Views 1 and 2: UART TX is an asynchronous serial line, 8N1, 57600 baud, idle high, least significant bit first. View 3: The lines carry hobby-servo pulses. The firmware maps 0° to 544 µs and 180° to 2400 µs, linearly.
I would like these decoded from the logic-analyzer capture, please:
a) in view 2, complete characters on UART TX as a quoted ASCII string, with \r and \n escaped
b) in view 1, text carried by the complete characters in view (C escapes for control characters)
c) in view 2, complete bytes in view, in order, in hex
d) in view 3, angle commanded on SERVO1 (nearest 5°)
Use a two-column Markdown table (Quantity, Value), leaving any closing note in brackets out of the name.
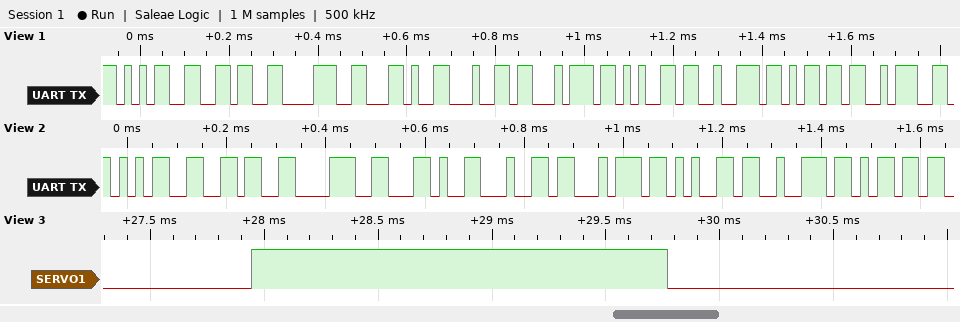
| Quantity | Value |
|---|---|
| in view 2, complete characters on UART TX as a quoted ASCII string, with \r and \n escaped | "568,dterm" |
| in view 1, text carried by the complete characters in view | "568,dterm:" |
| in view 2, complete bytes in view, in order, in hex | 35 36 38 2C 64 74 65 72 6D |
| in view 3, angle commanded on SERVO1 | 125° |
